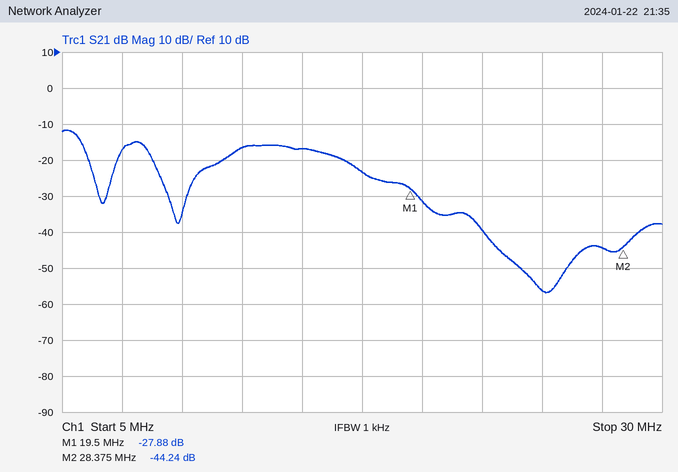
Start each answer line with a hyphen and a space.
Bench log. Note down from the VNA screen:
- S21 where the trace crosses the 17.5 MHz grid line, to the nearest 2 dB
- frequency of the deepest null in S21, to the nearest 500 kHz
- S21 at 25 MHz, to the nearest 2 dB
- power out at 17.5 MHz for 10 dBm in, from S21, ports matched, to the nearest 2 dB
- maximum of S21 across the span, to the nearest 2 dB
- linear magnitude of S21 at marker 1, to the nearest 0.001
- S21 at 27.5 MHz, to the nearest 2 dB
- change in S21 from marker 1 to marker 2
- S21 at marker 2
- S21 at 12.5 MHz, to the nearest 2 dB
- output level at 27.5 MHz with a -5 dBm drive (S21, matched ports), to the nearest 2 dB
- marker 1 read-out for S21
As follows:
- -24 dB
- 25.0 MHz
- -56 dB
- -14 dBm
- -12 dB
- 0.040
- -44 dB
- -16.36 dB
- -44.24 dB
- -16 dB
- -50 dBm
- -27.88 dB
